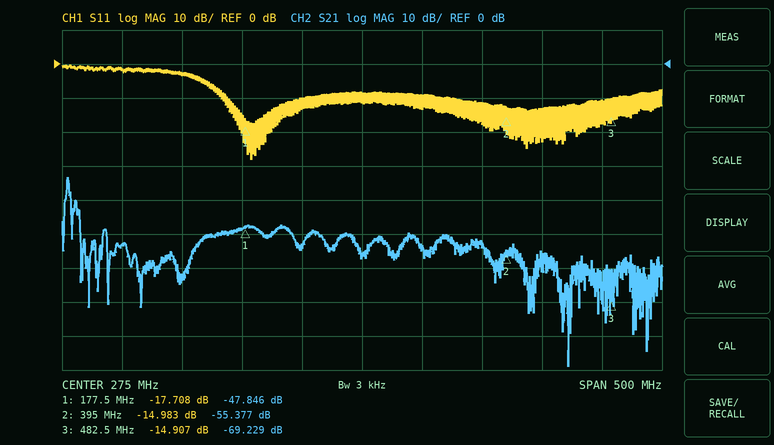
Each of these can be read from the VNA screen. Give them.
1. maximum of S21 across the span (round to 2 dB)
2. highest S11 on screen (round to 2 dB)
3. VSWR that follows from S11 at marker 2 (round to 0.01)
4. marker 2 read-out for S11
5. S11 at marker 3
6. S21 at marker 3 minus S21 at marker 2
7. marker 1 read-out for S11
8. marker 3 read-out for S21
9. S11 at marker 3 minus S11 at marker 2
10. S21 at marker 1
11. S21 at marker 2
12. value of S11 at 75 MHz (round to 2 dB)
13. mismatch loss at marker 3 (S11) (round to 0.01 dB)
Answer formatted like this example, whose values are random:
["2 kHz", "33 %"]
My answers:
["-34 dB", "0 dB", "1.43", "-14.983 dB", "-14.907 dB", "-13.852 dB", "-17.708 dB", "-69.229 dB", "0.076 dB", "-47.846 dB", "-55.377 dB", "-2 dB", "0.14 dB"]
